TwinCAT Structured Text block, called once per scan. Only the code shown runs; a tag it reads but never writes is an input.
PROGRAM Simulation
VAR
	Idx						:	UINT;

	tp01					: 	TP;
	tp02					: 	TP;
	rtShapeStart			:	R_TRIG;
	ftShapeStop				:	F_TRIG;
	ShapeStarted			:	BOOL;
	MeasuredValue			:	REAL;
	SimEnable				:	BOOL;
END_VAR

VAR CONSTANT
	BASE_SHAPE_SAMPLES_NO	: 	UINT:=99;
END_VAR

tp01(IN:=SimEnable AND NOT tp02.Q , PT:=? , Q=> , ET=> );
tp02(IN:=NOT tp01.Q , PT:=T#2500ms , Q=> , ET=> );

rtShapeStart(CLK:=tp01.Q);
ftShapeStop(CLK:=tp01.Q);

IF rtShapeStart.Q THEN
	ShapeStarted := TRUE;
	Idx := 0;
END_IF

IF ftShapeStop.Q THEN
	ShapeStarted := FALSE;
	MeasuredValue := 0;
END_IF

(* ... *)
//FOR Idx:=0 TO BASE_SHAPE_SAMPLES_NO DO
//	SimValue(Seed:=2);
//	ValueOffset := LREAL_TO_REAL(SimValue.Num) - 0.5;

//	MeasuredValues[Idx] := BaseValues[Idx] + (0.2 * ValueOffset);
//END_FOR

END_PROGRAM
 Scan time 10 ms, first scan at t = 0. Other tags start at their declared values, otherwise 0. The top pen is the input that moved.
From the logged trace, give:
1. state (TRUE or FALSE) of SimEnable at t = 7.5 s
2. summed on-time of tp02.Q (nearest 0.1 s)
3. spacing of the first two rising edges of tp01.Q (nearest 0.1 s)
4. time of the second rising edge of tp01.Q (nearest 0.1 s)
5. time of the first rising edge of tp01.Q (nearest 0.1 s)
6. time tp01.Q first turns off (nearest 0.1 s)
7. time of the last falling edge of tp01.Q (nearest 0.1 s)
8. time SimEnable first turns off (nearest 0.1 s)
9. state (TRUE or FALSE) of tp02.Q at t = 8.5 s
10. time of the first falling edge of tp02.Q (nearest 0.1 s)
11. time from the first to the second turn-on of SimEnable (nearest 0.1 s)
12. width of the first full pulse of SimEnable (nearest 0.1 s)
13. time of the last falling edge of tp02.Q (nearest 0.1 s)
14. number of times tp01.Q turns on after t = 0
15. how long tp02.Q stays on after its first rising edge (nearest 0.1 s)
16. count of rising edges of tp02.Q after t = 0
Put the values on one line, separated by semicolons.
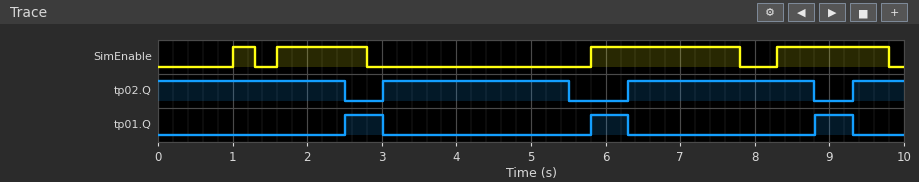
TRUE; 8.2 s; 3.3 s; 5.8 s; 2.5 s; 3.0 s; 9.3 s; 1.3 s; TRUE; 2.5 s; 0.6 s; 0.3 s; 8.8 s; 3; 2.5 s; 3
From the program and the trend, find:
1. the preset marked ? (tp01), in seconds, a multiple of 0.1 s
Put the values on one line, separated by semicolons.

0.5 s
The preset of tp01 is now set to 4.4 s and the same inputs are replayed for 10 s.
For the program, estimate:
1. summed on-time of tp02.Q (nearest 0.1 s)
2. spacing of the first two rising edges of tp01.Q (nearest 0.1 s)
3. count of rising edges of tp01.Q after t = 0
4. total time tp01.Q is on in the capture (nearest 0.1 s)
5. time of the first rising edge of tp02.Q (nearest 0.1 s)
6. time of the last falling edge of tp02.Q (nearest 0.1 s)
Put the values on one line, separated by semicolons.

5.0 s; 6.9 s; 2; 5.0 s; 6.9 s; 9.4 s
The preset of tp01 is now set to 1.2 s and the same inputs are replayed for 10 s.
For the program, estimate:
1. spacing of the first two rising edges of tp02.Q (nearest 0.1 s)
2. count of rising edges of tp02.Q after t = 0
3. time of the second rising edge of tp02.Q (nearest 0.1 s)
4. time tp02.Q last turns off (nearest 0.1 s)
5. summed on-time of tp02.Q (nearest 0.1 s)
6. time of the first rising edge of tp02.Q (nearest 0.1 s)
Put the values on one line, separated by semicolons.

3.7 s; 2; 7.4 s; 9.9 s; 7.5 s; 3.7 s
